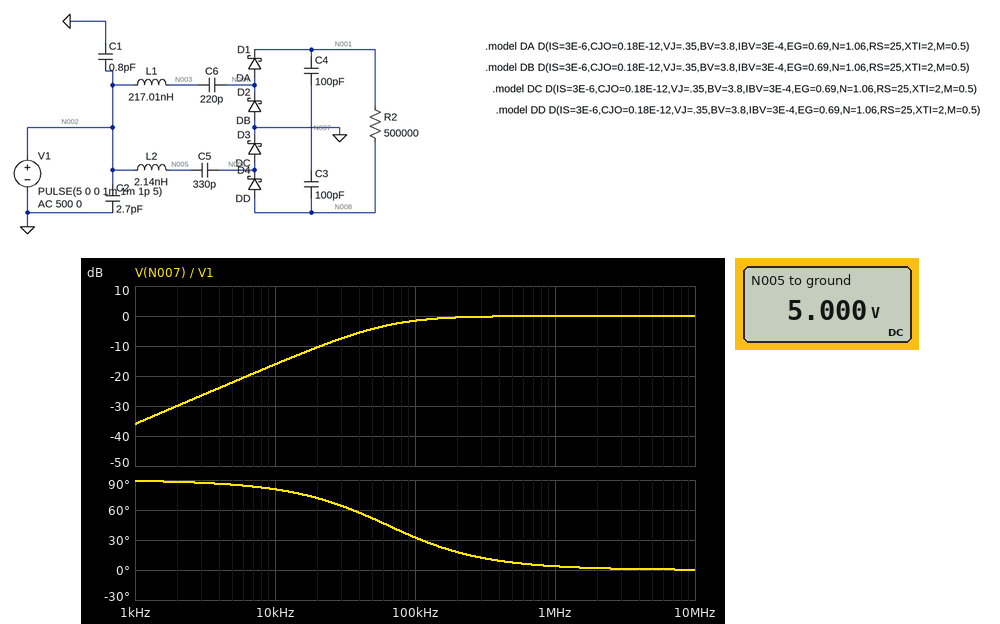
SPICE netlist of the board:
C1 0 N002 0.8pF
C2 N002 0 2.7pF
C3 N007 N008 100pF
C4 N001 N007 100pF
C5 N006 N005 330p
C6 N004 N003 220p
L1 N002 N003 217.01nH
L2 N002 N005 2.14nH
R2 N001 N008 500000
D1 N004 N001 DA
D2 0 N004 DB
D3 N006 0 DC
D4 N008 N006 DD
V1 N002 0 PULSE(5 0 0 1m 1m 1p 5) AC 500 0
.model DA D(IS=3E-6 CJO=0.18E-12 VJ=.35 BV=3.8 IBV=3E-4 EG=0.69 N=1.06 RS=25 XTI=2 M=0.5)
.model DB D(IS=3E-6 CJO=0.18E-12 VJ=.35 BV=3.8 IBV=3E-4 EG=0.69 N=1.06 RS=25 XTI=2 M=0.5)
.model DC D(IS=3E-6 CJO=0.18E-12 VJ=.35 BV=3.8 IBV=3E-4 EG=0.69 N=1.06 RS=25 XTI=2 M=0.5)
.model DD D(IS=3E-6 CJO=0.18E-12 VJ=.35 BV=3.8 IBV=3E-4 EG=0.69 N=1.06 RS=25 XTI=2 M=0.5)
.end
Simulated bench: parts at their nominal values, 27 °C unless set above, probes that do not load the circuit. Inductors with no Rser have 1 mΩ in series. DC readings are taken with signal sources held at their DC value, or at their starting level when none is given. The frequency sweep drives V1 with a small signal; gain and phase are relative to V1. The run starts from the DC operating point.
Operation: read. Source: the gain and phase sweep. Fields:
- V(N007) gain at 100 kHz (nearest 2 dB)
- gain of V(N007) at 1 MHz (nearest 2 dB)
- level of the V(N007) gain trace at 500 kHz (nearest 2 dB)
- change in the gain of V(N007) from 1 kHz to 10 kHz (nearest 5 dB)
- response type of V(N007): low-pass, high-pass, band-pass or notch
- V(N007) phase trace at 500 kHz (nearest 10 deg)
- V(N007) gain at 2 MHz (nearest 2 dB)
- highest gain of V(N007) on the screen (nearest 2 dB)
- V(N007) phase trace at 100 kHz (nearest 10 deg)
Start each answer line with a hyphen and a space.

- -2 dB
- 0 dB
- 0 dB
- 20 dB
- high-pass
- 10 deg
- 0 dB
- 0 dB
- 30 deg
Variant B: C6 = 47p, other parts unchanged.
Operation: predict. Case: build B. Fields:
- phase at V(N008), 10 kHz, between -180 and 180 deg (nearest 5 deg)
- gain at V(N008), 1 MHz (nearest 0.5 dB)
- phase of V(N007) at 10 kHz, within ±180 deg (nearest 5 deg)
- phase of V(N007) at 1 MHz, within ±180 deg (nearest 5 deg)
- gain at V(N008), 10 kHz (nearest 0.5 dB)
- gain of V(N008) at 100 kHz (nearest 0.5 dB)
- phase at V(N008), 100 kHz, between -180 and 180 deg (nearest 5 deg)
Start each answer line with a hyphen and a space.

- 75 deg
- -0.5 dB
- 80 deg
- 10 deg
- -15.0 dB
- -3.0 dB
- 25 deg
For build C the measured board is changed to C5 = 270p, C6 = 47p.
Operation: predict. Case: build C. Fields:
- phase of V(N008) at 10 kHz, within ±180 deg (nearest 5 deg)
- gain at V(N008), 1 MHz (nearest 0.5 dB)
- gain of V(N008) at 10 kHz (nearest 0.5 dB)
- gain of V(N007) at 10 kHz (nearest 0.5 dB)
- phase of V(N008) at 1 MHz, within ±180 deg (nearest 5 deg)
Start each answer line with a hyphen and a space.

- 80 deg
- -0.5 dB
- -16.5 dB
- -21.0 dB
- 10 deg
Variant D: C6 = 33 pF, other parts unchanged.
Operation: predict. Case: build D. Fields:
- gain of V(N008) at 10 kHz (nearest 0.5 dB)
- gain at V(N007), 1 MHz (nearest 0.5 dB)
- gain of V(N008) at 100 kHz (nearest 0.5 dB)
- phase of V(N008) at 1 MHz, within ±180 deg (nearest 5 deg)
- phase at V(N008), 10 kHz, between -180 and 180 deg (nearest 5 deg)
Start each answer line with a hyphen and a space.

- -15.0 dB
- -1.0 dB
- -3.0 dB
- 10 deg
- 75 deg
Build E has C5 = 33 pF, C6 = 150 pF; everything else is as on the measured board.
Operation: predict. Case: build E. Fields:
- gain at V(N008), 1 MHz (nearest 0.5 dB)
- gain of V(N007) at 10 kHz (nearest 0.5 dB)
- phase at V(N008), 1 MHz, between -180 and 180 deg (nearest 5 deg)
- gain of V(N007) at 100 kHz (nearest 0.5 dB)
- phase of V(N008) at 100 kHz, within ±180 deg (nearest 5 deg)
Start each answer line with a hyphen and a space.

- -0.5 dB
- -25.5 dB
- 15 deg
- -7.5 dB
- 80 deg
